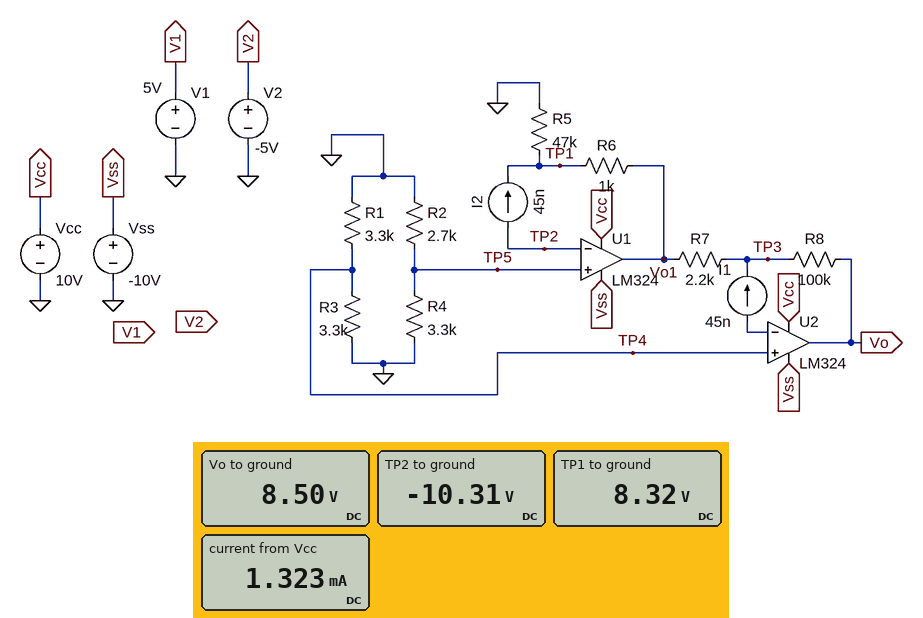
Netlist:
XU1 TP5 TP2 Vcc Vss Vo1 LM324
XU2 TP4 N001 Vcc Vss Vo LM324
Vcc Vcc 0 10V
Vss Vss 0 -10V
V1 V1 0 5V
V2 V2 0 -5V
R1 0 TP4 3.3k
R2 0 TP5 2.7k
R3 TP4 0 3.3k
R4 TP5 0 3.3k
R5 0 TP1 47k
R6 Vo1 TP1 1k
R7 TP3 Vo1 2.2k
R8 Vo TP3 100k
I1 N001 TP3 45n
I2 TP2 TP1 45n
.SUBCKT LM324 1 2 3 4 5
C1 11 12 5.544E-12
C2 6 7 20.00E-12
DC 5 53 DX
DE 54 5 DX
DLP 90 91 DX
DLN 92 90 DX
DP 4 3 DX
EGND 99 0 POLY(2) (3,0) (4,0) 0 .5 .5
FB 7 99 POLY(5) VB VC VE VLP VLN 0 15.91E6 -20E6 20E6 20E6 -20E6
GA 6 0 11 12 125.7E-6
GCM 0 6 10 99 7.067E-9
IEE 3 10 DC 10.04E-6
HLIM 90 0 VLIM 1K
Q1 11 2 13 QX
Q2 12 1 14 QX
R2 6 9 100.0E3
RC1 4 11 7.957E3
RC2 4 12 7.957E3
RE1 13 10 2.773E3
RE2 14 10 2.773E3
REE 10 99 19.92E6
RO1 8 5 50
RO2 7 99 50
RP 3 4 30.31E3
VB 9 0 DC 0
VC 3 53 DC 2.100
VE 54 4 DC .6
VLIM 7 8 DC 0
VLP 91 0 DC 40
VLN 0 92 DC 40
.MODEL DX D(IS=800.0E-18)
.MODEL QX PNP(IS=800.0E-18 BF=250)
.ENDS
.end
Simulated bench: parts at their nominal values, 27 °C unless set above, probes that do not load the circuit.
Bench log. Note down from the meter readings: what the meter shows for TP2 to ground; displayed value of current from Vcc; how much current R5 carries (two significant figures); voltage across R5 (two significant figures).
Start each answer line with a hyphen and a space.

- -10.31 V
- 1.323 mA
- 180 µA
- 8.3 V
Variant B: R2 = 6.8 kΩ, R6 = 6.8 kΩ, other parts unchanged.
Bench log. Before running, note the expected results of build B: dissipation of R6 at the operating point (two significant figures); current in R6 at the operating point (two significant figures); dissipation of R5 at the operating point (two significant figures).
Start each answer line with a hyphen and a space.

- 170 µW
- 160 µA
- 1.2 mW
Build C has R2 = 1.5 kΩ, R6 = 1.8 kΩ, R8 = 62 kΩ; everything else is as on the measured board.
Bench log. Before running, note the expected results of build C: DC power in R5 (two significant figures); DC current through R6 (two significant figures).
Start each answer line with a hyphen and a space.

- 1.4 mW
- 170 µA
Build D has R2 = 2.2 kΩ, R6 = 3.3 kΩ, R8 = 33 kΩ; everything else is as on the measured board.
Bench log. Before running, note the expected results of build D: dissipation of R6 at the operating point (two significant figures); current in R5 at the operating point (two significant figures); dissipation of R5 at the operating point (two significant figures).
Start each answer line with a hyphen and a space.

- 94 µW
- 170 µA
- 1.3 mW
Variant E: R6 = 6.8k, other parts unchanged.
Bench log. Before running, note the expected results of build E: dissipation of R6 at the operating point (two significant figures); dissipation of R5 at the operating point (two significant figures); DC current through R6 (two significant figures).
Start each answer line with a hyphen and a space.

- 170 µW
- 1.2 mW
- 160 µA
